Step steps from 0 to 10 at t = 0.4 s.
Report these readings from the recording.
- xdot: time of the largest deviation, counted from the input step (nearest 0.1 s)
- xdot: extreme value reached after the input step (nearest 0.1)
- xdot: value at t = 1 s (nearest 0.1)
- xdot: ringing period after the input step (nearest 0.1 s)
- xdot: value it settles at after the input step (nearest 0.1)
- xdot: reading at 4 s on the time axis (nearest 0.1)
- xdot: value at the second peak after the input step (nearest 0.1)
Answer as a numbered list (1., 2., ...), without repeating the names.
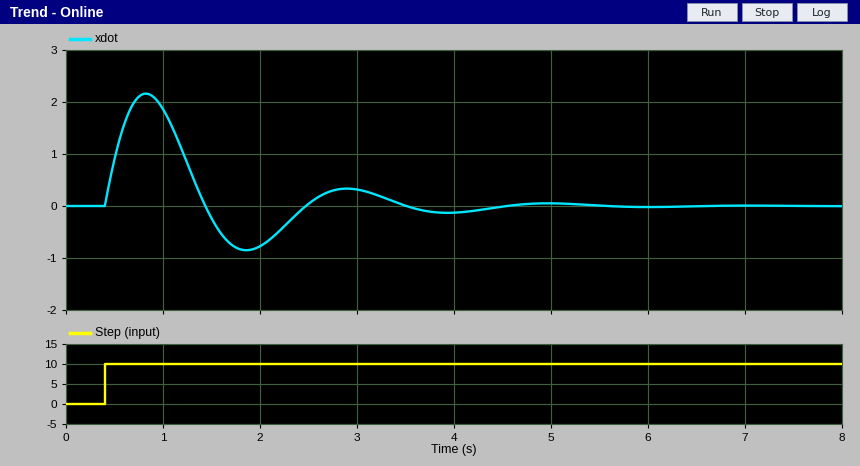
1. 0.4 s
2. 2.2
3. 1.9
4. 2.1 s
5. 0.0
6. -0.1
7. 0.3
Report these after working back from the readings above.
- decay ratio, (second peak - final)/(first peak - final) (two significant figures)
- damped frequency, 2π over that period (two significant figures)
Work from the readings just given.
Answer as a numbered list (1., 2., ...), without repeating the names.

1. 0.14
2. 3.0 rad/s
